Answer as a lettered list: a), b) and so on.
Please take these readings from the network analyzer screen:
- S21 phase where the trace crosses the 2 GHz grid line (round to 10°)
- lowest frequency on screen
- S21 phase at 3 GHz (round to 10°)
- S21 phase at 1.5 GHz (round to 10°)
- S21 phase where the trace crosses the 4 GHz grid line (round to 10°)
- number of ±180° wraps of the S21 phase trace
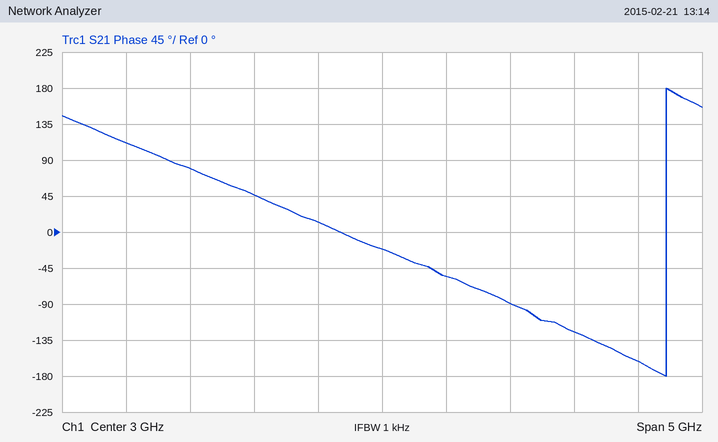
a) 50°
b) 500 MHz
c) -20°
d) 80°
e) -90°
f) 1
